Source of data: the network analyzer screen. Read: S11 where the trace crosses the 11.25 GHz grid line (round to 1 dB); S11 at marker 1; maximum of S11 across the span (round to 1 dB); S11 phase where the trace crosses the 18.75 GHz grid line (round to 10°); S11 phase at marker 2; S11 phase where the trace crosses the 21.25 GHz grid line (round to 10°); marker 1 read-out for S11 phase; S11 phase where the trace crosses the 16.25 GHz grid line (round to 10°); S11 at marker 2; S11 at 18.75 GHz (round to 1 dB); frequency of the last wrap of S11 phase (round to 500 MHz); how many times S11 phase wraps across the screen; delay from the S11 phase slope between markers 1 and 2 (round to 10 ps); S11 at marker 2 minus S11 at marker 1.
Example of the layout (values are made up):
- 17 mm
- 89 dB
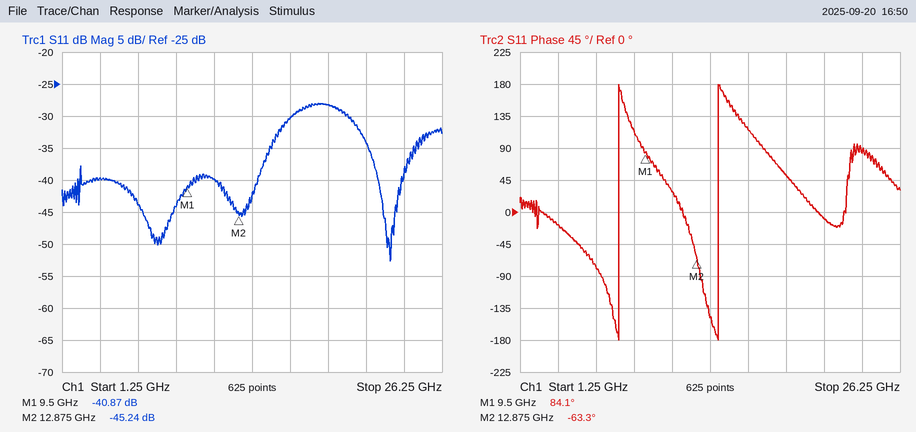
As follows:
- -40 dB
- -40.87 dB
- -28 dB
- 50°
- -63.3°
- -10°
- 84.1°
- 120°
- -45.24 dB
- -28 dB
- 14.5 GHz
- 2
- 120 ps
- -4.37 dB
